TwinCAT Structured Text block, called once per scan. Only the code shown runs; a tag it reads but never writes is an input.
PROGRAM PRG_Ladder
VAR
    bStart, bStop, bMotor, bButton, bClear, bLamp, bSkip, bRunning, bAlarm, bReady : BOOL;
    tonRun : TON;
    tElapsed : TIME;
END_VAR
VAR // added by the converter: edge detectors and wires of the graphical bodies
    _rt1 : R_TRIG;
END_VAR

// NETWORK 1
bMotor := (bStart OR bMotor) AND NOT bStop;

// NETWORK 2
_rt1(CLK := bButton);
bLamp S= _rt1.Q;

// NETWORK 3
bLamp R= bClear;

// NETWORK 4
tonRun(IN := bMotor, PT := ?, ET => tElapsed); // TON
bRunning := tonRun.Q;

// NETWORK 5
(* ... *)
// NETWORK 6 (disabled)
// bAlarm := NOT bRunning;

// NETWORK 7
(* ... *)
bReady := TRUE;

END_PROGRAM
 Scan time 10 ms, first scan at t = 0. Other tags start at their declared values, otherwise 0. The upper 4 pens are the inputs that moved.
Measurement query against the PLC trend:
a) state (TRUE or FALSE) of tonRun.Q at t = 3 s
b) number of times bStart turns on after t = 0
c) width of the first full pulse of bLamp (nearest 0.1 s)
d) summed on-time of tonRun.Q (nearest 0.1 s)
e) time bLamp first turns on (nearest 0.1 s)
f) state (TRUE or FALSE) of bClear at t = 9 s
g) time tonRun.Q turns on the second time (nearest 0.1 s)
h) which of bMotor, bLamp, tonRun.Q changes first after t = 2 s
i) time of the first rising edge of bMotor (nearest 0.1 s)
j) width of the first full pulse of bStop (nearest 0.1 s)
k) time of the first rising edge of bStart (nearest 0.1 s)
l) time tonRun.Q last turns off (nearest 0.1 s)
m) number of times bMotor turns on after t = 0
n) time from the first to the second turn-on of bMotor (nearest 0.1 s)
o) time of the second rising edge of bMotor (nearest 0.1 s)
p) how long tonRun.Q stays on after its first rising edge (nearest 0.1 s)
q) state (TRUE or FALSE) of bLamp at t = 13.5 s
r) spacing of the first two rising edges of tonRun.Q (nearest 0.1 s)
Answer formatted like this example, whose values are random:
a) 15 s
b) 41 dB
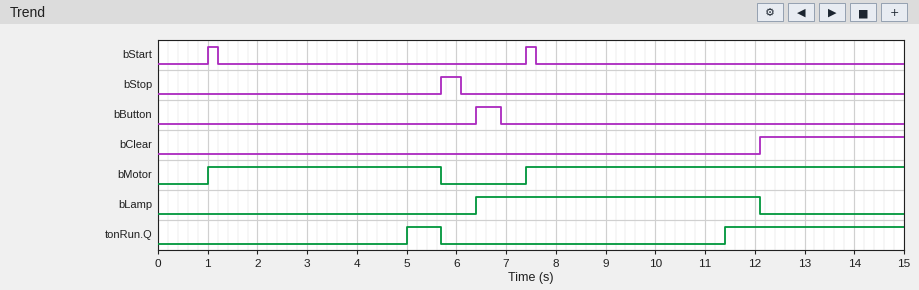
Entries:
a) FALSE
b) 2
c) 5.7 s
d) 4.3 s
e) 6.4 s
f) FALSE
g) 11.4 s
h) tonRun.Q
i) 1.0 s
j) 0.4 s
k) 1.0 s
l) 5.7 s
m) 2
n) 6.4 s
o) 7.4 s
p) 0.7 s
q) FALSE
r) 6.4 s
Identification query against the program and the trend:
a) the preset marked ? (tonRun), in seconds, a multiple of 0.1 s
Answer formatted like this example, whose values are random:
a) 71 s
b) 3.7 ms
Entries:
a) 4.0 s
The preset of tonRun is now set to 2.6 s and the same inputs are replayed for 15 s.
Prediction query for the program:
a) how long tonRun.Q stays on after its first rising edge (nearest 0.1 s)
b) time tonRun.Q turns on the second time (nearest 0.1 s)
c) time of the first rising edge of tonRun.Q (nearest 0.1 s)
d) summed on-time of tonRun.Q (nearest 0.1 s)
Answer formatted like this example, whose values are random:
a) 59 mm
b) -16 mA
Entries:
a) 2.1 s
b) 10.0 s
c) 3.6 s
d) 7.1 s
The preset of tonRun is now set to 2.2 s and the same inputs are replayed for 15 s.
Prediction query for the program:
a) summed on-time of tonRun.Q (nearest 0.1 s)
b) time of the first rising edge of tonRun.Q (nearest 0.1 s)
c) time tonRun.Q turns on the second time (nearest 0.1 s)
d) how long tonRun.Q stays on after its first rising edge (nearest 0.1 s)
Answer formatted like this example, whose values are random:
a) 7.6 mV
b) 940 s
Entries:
a) 7.9 s
b) 3.2 s
c) 9.6 s
d) 2.5 s
